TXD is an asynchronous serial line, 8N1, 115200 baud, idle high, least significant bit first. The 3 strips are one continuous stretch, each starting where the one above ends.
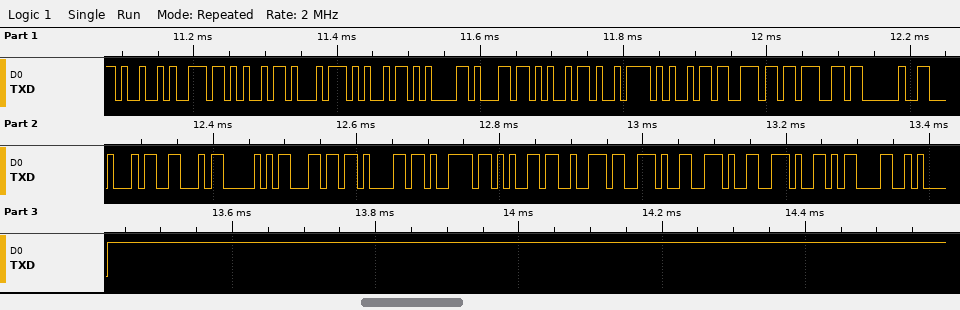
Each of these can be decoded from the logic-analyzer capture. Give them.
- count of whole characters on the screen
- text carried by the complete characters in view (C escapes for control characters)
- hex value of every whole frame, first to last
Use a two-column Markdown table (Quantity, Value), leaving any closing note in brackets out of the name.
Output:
| Quantity | Value |
|---|---|
| count of whole characters on the screen | 26 |
| text carried by the complete characters in view | "Initializing DFPlayer...\r\n" |
| hex value of every whole frame, first to last | 0x49 0x6E 0x69 0x74 0x69 0x61 0x6C 0x69 0x7A 0x69 0x6E 0x67 0x20 0x44 0x46 0x50 0x6C 0x61 0x79 0x65 0x72 0x2E 0x2E 0x2E 0x0D 0x0A |
